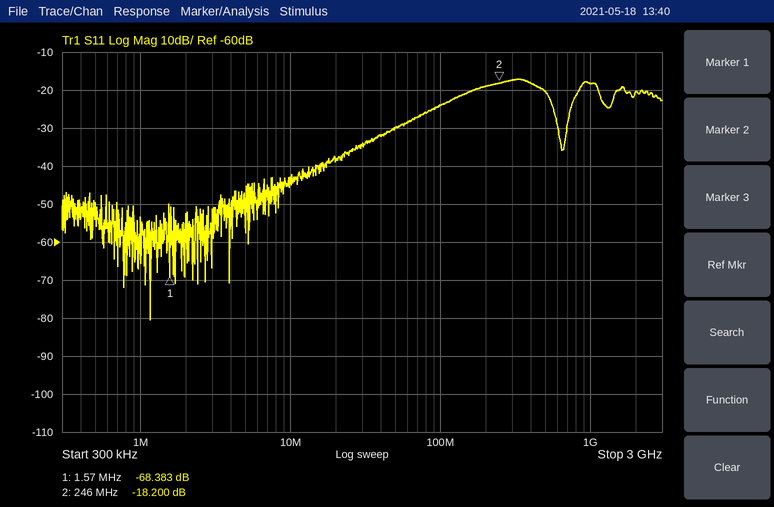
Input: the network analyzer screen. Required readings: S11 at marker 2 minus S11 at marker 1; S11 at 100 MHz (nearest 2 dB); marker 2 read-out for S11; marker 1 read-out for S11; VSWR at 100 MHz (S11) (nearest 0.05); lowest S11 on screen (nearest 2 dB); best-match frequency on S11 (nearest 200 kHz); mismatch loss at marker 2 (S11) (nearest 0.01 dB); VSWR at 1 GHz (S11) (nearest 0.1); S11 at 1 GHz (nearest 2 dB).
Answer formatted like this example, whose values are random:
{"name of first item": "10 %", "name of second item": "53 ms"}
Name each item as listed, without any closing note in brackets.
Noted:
{"S11 at marker 2 minus S11 at marker 1": "50.183 dB", "S11 at 100 MHz": "-24 dB", "marker 2 read-out for S11": "-18.200 dB", "marker 1 read-out for S11": "-68.383 dB", "VSWR at 100 MHz (S11)": "1.15", "lowest S11 on screen": "-80 dB", "best-match frequency on S11": "1.2 MHz", "mismatch loss at marker 2 (S11)": "0.07 dB", "VSWR at 1 GHz (S11)": "1.3", "S11 at 1 GHz": "-18 dB"}
